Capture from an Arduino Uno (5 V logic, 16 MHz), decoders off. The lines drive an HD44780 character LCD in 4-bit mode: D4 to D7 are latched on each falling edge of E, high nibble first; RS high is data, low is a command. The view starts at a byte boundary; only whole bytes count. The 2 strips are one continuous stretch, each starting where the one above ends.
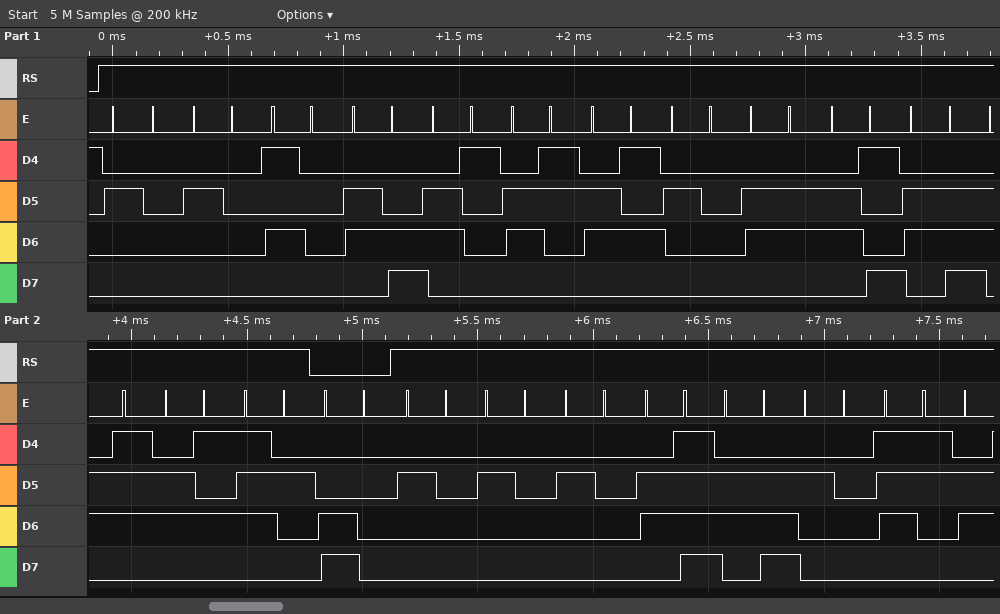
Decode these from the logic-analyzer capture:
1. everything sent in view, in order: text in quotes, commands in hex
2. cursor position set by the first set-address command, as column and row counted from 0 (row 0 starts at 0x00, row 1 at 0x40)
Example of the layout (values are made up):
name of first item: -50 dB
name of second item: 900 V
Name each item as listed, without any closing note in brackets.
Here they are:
everything sent in view, in order: text in quotes, commands in hex: "  Place finger" 0xC0 "   on s"
cursor position set by the first set-address command, as column and row counted from 0: column 0, row 1
